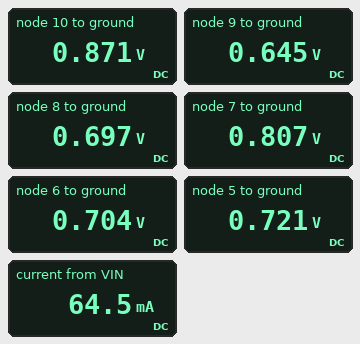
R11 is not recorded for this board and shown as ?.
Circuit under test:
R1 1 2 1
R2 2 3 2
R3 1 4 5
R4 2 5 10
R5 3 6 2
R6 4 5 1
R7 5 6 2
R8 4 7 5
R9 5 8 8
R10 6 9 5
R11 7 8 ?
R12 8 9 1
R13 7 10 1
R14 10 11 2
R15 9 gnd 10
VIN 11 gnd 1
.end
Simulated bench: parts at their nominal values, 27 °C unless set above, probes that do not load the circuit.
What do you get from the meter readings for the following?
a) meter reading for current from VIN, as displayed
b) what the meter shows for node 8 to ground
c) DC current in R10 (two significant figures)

64.5 mA
0.697 V
12 mA
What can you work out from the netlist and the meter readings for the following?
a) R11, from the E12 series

2.2 Ω
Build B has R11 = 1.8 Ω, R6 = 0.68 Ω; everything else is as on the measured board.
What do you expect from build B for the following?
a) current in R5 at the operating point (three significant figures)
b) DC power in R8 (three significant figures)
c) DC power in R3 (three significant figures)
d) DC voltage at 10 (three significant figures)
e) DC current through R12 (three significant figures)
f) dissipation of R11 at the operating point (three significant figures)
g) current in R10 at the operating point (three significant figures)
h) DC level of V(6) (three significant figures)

2.79 mA
912 µW
24.7 µW
869 mV
54.3 mA
4.87 mW
11.2 mA
711 mV
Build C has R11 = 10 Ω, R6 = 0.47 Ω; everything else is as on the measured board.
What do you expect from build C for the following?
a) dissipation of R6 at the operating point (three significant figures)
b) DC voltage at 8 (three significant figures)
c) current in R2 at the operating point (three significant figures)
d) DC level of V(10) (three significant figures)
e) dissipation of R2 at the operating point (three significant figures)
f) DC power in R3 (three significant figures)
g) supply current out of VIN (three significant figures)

324 µW
585 mV
4.69 mA
890 mV
44.0 µW
68.5 µW
54.9 mA
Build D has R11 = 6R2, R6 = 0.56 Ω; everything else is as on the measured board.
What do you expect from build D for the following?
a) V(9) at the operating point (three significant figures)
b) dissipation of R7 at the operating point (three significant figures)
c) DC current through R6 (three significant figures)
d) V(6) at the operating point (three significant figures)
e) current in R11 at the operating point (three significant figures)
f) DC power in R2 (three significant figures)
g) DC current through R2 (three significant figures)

580 mV
311 µW
21.7 mA
664 mV
33.0 mA
35.3 µW
4.20 mA
